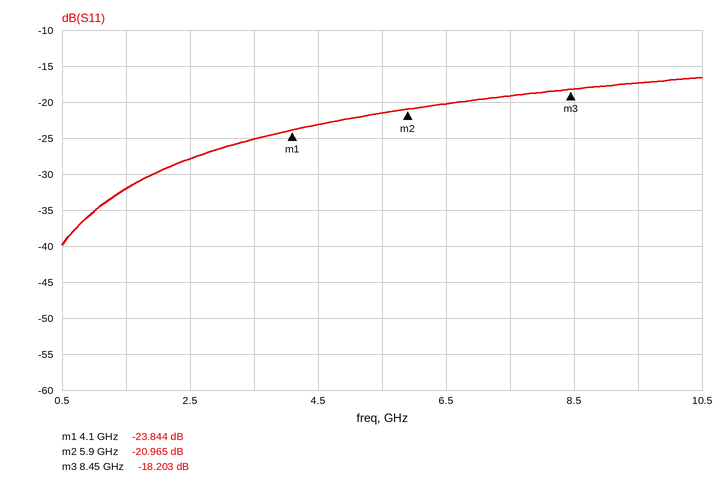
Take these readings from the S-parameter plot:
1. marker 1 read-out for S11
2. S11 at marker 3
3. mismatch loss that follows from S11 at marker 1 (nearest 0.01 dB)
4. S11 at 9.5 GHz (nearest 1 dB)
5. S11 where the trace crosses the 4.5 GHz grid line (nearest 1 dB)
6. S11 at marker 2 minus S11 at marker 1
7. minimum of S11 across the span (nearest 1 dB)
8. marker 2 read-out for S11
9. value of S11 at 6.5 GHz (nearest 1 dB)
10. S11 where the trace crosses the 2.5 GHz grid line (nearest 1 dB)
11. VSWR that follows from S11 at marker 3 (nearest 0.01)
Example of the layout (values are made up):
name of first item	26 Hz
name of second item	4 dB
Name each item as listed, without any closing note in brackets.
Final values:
marker 1 read-out for S11	-23.844 dB
S11 at marker 3	-18.203 dB
mismatch loss that follows from S11 at marker 1	0.02 dB
S11 at 9.5 GHz	-17 dB
S11 where the trace crosses the 4.5 GHz grid line	-23 dB
S11 at marker 2 minus S11 at marker 1	2.879 dB
minimum of S11 across the span	-40 dB
marker 2 read-out for S11	-20.965 dB
value of S11 at 6.5 GHz	-20 dB
S11 where the trace crosses the 2.5 GHz grid line	-28 dB
VSWR that follows from S11 at marker 3	1.28
